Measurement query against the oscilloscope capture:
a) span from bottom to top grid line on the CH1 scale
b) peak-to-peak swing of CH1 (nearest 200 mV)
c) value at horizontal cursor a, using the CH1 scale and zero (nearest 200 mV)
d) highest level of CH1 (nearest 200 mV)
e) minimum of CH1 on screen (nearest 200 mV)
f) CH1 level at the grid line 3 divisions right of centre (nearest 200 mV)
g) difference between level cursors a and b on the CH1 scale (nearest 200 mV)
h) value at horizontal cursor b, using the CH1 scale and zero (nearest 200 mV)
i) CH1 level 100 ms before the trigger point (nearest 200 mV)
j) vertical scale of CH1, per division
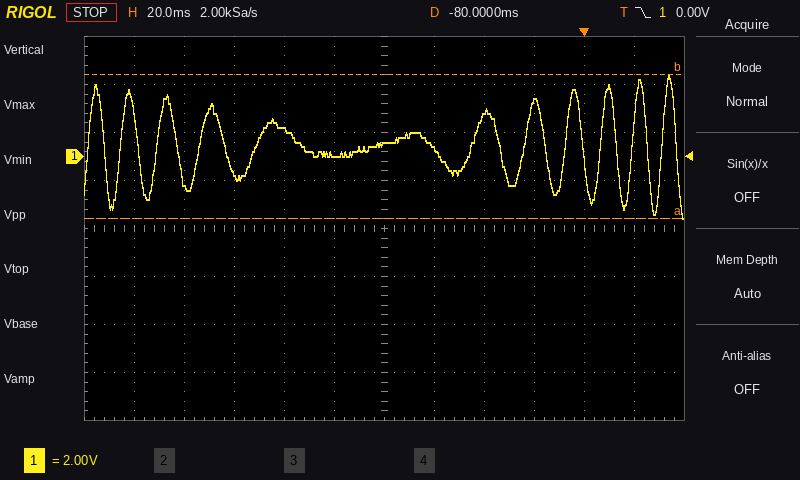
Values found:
16 V
6.0 V
-2.6 V
3.4 V
-2.6 V
2.2 V
6.0 V
3.4 V
0.0 V
2 V
